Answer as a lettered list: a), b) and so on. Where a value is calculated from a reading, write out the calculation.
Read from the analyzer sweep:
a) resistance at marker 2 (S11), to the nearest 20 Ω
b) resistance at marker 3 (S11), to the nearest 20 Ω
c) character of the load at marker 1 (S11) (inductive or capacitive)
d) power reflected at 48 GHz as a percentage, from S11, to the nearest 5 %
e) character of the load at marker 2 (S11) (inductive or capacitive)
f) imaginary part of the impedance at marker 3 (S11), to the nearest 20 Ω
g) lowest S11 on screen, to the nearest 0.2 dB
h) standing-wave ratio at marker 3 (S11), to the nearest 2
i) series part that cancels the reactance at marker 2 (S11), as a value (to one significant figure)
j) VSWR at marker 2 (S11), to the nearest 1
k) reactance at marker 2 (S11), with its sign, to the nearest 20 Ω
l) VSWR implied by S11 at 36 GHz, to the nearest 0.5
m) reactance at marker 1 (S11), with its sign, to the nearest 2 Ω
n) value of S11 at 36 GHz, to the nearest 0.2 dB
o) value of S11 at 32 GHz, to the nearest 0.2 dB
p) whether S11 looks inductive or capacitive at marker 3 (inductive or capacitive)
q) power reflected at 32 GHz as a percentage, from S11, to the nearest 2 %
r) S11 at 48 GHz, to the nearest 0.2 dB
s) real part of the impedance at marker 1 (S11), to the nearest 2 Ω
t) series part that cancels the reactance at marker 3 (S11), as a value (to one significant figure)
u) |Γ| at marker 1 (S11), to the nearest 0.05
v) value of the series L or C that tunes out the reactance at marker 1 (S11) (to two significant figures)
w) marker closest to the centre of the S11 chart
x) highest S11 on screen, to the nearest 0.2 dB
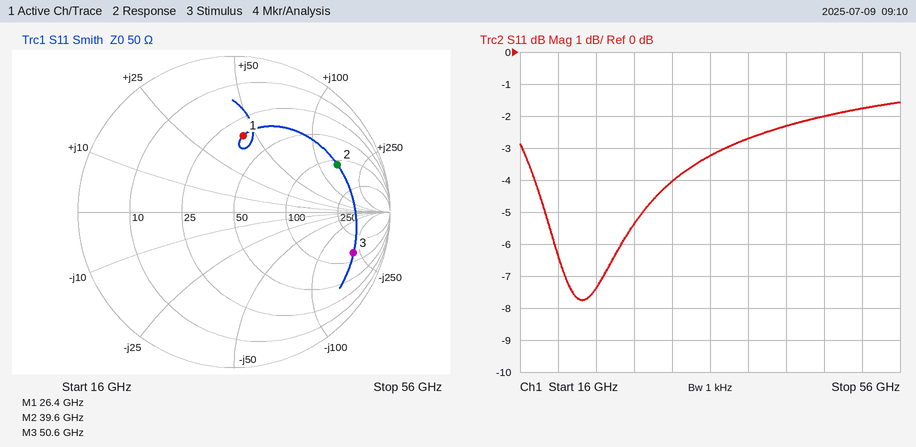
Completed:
a) 120 Ω
b) 140 Ω
c) inductive
d) 10^(-2/10) ≈ 63.1 %, so 65 % to the nearest 5 %
e) inductive
f) -220 Ω
g) -7.8 dB
h) 10
i) C = 1/(2π × 39.6 GHz × 140 Ω) ≈ 28.7 fF, so 30 fF to one significant figure
j) 6
k) +140 Ω
l) |Γ| = 10^(-3.2/20) = 0.6918; VSWR = (1 + 0.6918)/(1 − 0.6918) ≈ 5.5
m) +44 Ω
n) -3.2 dB
o) -4.0 dB
p) capacitive
q) 10^(-4/10) ≈ 40 %
r) -2.0 dB
s) 34 Ω
t) L = 220 Ω/(2π × 50.6 GHz) ≈ 692 pH, so 700 pH to one significant figure
u) 0.50
v) C = 1/(2π × 26.4 GHz × 44 Ω) ≈ 137 fF, so 140 fF to two significant figures
w) marker 1
x) -1.6 dB
